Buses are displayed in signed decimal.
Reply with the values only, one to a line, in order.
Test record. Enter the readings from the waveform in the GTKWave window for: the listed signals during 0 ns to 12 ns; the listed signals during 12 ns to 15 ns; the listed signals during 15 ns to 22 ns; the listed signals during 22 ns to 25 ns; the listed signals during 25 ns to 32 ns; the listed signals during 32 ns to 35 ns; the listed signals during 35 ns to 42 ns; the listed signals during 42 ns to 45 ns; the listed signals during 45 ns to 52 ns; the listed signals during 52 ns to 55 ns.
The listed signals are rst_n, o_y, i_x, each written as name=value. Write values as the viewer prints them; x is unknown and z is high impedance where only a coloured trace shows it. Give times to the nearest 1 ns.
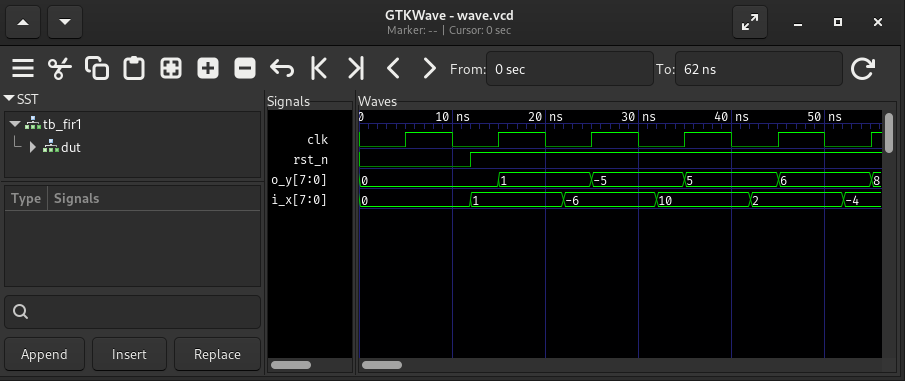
rst_n=0, o_y=0, i_x=0
rst_n=1, o_y=0, i_x=1
rst_n=1, o_y=1, i_x=1
rst_n=1, o_y=1, i_x=-6
rst_n=1, o_y=-5, i_x=-6
rst_n=1, o_y=-5, i_x=10
rst_n=1, o_y=5, i_x=10
rst_n=1, o_y=5, i_x=2
rst_n=1, o_y=6, i_x=2
rst_n=1, o_y=6, i_x=-4
